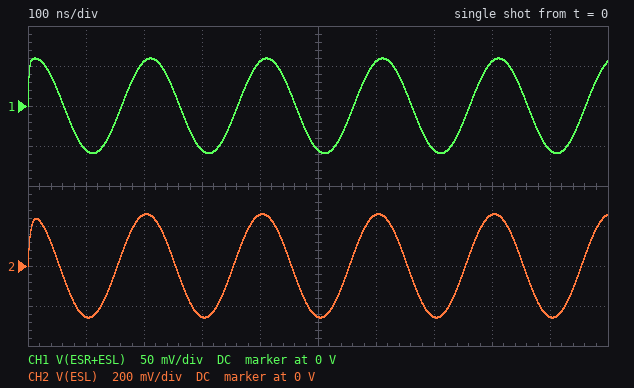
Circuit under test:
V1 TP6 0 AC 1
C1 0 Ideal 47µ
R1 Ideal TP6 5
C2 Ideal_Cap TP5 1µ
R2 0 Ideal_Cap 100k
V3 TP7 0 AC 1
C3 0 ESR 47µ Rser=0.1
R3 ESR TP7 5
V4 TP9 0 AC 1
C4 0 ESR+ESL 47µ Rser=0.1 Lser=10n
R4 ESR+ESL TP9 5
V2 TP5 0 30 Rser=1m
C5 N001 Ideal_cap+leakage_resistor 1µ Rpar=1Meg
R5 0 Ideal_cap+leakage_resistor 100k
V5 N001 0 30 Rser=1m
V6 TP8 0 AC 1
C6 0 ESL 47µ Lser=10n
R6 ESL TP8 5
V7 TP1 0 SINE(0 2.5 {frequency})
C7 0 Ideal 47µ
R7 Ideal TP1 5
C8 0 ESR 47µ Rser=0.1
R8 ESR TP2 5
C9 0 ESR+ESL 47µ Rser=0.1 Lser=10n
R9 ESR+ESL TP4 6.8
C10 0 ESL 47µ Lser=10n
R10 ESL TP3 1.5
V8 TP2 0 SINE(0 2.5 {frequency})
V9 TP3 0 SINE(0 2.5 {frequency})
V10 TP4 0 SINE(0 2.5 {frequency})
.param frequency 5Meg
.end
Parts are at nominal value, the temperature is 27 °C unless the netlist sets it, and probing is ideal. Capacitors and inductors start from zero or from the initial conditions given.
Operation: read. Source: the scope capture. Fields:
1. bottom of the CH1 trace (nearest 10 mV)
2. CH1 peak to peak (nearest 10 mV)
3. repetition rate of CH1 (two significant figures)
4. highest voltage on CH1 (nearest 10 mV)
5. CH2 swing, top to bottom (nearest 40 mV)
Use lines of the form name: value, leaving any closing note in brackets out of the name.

bottom of the CH1 trace: -60 mV
CH1 peak to peak: 120 mV
repetition rate of CH1: 5.0 MHz
highest voltage on CH1: 60 mV
CH2 swing, top to bottom: 520 mV
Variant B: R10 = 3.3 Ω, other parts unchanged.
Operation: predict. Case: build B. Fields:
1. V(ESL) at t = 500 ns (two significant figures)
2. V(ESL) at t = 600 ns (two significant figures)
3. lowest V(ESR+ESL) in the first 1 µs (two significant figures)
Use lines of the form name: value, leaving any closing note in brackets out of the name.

V(ESL) at t = 500 ns: -120 mV
V(ESL) at t = 600 ns: 120 mV
lowest V(ESR+ESL) in the first 1 µs: -59 mV
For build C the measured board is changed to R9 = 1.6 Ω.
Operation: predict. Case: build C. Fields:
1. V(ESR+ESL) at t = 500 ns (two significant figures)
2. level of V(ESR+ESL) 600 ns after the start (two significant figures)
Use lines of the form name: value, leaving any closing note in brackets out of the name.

V(ESR+ESL) at t = 500 ns: -220 mV
level of V(ESR+ESL) 600 ns after the start: 220 mV
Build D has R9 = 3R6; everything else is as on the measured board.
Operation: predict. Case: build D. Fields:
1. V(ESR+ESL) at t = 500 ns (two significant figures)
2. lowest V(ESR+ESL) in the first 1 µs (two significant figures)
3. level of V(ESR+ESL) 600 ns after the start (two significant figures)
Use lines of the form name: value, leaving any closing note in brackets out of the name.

V(ESR+ESL) at t = 500 ns: -100 mV
lowest V(ESR+ESL) in the first 1 µs: -110 mV
level of V(ESR+ESL) 600 ns after the start: 100 mV
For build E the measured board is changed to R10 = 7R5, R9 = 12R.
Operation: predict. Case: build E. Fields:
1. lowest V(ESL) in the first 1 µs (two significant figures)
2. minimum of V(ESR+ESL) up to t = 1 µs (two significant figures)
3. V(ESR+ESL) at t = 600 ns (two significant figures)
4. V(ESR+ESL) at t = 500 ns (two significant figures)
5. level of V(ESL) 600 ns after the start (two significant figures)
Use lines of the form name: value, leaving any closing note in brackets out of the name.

lowest V(ESL) in the first 1 µs: -52 mV
minimum of V(ESR+ESL) up to t = 1 µs: -34 mV
V(ESR+ESL) at t = 600 ns: 32 mV
V(ESR+ESL) at t = 500 ns: -32 mV
level of V(ESL) 600 ns after the start: 52 mV
